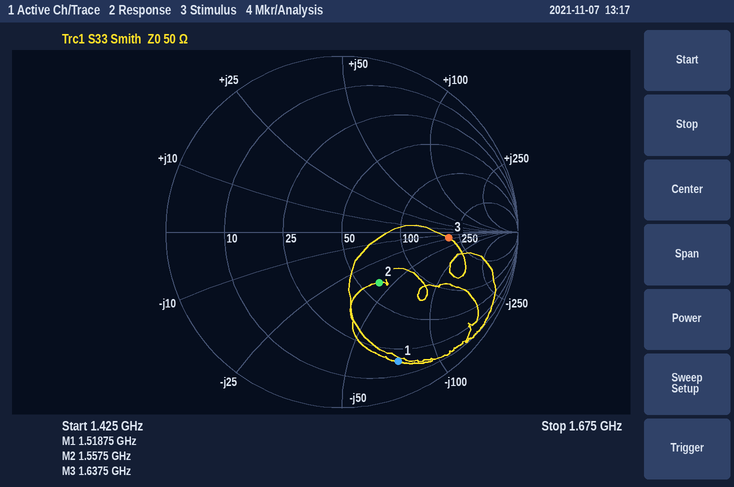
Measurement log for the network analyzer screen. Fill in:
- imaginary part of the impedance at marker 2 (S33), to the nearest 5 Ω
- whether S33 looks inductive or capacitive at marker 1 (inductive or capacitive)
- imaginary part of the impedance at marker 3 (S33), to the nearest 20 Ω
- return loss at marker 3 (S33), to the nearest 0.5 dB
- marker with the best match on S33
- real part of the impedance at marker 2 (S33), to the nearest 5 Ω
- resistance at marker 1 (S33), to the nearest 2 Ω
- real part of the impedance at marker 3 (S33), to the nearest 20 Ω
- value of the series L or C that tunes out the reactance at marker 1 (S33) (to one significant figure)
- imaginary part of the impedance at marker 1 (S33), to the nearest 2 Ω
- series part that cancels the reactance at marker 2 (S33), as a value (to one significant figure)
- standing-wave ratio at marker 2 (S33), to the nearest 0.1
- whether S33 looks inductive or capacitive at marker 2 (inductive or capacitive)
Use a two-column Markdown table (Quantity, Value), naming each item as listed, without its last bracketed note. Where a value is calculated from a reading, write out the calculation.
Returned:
| Quantity | Value |
|---|---|
| imaginary part of the impedance at marker 2 (S33), to the nearest 5 Ω | -40 Ω |
| whether S33 looks inductive or capacitive at marker 1 | capacitive |
| imaginary part of the impedance at marker 3 (S33), to the nearest 20 Ω | -20 Ω |
| return loss at marker 3 (S33), to the nearest 0.5 dB | 4.5 dB |
| marker with the best match on S33 | marker 2 |
| real part of the impedance at marker 2 (S33), to the nearest 5 Ω | 60 Ω |
| resistance at marker 1 (S33), to the nearest 2 Ω | 18 Ω |
| real part of the impedance at marker 3 (S33), to the nearest 20 Ω | 200 Ω |
| value of the series L or C that tunes out the reactance at marker 1 (S33) | L = 74 Ω/(2π × 1.51875 GHz) ≈ 8 nH |
| imaginary part of the impedance at marker 1 (S33), to the nearest 2 Ω | -74 Ω |
| series part that cancels the reactance at marker 2 (S33), as a value | L = 40 Ω/(2π × 1.5575 GHz) ≈ 4 nH |
| standing-wave ratio at marker 2 (S33), to the nearest 0.1 | 2.1 |
| whether S33 looks inductive or capacitive at marker 2 | capacitive |
